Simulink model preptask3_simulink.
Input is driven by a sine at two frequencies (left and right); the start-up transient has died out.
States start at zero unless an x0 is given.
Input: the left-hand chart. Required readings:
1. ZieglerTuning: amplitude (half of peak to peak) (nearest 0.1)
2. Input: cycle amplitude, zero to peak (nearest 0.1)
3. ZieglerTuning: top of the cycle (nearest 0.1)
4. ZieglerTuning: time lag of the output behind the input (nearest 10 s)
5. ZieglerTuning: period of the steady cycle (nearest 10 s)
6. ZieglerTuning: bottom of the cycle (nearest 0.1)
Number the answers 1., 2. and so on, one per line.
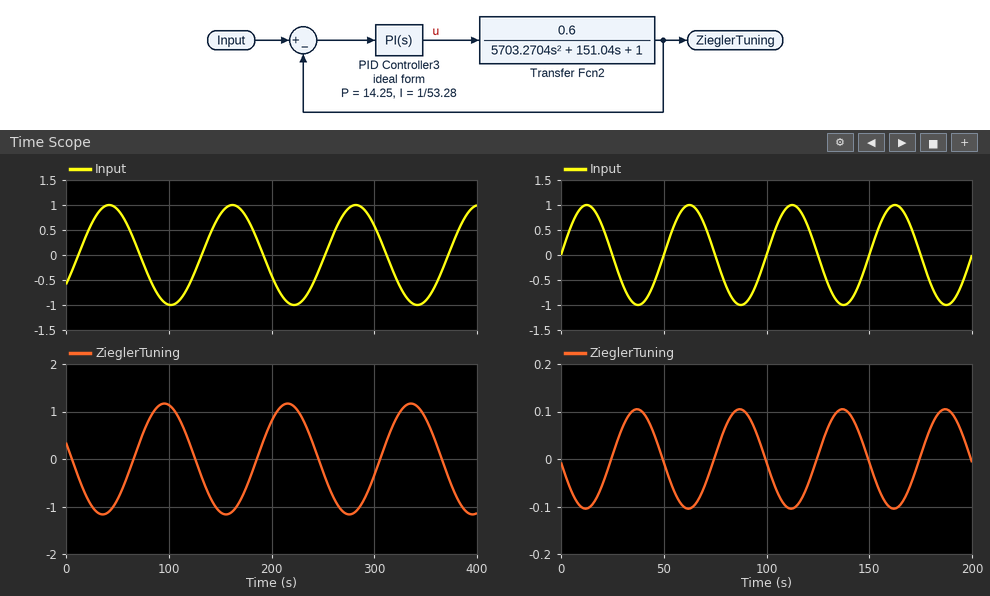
1. 1.2
2. 1.0
3. 1.2
4. 50 s
5. 120 s
6. -1.2
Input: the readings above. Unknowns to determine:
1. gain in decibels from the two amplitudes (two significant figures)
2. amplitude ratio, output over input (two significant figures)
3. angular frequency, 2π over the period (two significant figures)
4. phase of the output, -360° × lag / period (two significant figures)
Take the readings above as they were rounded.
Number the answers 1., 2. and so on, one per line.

1. 1.6 dB
2. 1.2
3. 0.052 rad/s
4. -150°
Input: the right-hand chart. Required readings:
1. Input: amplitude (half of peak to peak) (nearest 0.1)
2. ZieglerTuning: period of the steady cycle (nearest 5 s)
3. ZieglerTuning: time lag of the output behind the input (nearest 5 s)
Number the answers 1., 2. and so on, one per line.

1. 1.0
2. 50 s
3. 25 s
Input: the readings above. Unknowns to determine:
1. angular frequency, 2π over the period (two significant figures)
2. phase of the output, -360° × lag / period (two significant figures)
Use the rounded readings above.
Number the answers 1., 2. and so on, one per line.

1. 0.13 rad/s
2. -180°
